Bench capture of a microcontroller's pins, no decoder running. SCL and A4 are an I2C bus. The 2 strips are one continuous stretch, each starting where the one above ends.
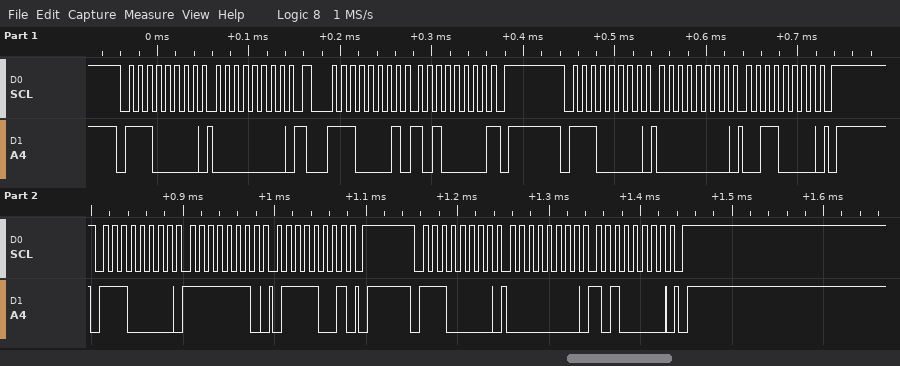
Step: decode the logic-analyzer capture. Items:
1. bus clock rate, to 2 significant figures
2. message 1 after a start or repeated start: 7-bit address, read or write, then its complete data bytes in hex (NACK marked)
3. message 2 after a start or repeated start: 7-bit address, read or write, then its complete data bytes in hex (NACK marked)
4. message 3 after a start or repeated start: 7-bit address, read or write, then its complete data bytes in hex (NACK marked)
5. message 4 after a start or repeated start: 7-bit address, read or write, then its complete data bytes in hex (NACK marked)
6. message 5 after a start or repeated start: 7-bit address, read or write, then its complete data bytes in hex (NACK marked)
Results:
100 kHz
0x70 write: 00
0x70 read: A0 NACK
0x70 write: 00 30
0x70 write: FE 79
0x70 write: 00 A0
